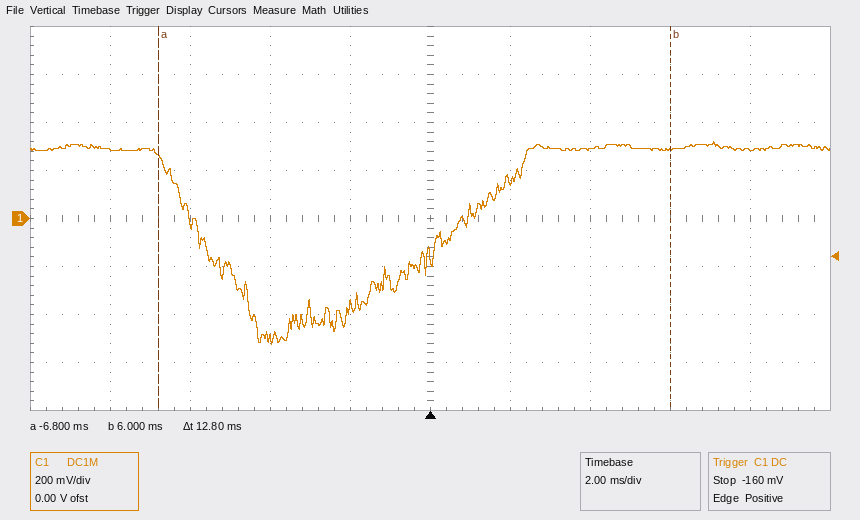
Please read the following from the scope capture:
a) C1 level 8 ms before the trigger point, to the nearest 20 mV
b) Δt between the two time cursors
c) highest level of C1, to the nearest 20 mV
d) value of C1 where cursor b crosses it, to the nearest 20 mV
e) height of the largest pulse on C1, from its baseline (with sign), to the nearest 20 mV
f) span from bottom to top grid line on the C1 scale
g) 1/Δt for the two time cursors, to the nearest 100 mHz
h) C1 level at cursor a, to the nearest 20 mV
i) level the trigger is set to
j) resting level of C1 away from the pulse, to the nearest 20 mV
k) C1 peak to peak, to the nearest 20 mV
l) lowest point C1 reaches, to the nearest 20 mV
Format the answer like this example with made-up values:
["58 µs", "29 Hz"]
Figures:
["280 mV", "12.8 ms", "320 mV", "280 mV", "-820 mV", "1.6 V", "78.1 Hz", "260 mV", "-160 mV", "300 mV", "840 mV", "-520 mV"]
